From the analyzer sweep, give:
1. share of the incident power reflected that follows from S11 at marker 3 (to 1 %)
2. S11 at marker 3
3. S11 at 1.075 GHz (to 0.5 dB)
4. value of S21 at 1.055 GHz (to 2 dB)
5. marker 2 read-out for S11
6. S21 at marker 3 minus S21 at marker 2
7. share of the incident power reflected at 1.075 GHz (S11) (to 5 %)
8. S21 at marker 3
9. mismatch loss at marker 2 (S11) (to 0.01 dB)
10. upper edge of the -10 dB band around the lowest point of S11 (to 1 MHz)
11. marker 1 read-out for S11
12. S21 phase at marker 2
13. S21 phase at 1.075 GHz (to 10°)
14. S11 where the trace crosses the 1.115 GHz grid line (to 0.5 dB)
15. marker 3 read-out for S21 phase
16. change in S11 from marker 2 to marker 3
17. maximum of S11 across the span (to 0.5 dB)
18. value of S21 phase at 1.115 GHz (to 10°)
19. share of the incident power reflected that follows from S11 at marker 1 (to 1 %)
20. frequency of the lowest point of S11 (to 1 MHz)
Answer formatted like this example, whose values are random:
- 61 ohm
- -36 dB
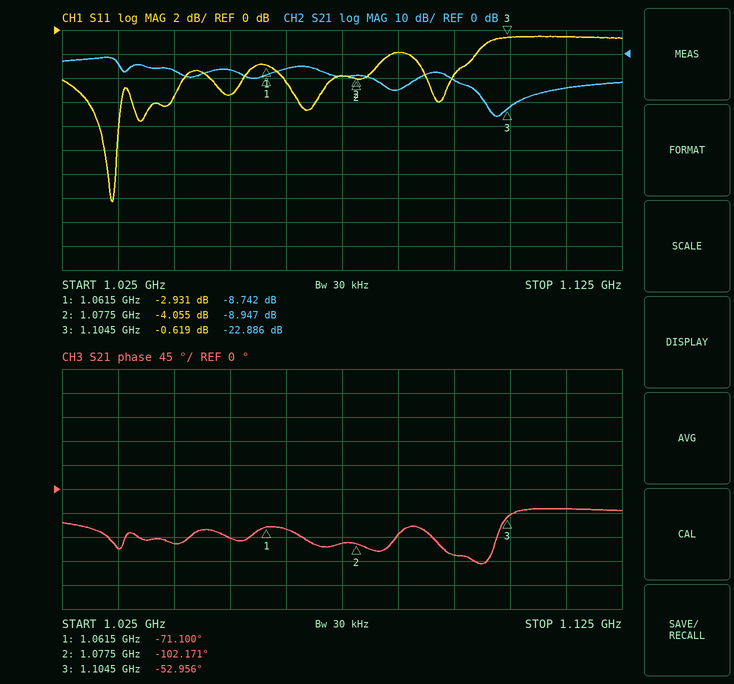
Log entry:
- 87 %
- -0.619 dB
- -4.0 dB
- -6 dB
- -4.055 dB
- -13.939 dB
- 40 %
- -22.886 dB
- 2.17 dB
- 1.035 GHz
- -2.931 dB
- -102.171°
- -100°
- -0.5 dB
- -52.956°
- 3.436 dB
- -0.5 dB
- -40°
- 51 %
- 1.034 GHz
